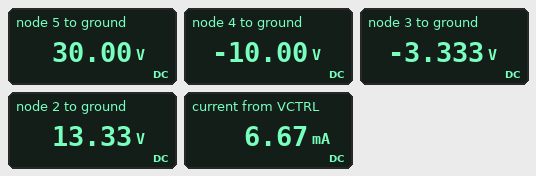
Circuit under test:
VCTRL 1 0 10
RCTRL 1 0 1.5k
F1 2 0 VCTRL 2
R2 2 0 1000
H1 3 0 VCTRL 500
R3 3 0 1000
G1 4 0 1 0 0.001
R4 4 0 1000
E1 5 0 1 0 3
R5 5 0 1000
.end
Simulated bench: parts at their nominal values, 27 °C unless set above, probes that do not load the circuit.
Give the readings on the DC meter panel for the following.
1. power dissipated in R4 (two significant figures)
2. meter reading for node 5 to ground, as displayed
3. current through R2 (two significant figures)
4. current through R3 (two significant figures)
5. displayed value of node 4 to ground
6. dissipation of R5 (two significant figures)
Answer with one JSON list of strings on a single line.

["100 mW", "30.00 V", "13 mA", "3.3 mA", "-10.00 V", "900 mW"]
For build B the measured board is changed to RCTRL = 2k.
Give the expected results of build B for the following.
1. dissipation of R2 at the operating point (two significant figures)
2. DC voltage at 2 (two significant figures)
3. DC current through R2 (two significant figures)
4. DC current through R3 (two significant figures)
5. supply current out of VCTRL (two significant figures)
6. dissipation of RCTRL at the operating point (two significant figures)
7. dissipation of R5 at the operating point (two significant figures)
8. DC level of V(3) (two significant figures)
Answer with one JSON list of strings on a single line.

["100 mW", "10 V", "10 mA", "2.5 mA", "5.0 mA", "50 mW", "900 mW", "-2.5 V"]
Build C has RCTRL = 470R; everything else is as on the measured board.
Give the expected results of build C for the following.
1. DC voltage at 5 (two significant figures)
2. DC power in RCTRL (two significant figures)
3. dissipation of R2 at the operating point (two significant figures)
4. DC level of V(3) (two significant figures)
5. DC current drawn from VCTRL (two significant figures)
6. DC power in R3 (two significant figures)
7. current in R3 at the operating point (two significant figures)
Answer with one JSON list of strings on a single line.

["30 V", "210 mW", "1.8 W", "-11 V", "21 mA", "110 mW", "11 mA"]
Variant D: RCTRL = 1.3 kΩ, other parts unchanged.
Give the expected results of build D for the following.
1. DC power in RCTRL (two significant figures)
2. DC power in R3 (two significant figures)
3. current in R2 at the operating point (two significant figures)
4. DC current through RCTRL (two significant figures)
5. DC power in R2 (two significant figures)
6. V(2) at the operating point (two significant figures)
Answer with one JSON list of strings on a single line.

["77 mW", "15 mW", "15 mA", "7.7 mA", "240 mW", "15 V"]
